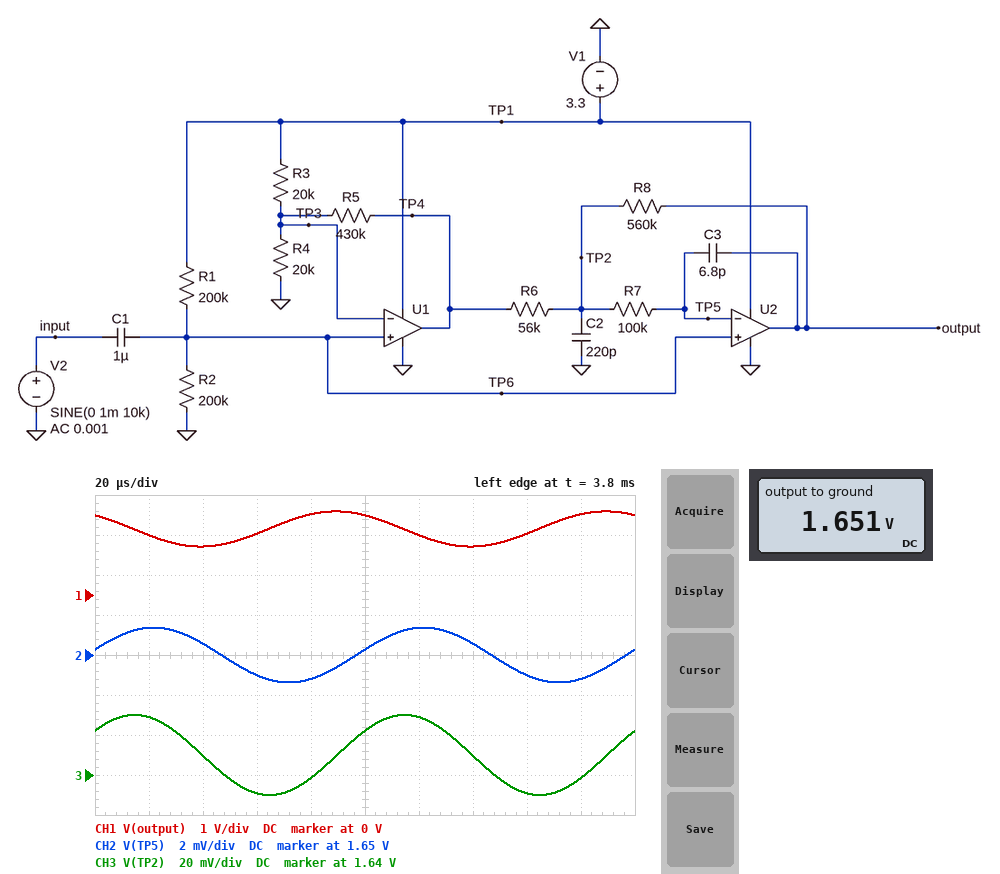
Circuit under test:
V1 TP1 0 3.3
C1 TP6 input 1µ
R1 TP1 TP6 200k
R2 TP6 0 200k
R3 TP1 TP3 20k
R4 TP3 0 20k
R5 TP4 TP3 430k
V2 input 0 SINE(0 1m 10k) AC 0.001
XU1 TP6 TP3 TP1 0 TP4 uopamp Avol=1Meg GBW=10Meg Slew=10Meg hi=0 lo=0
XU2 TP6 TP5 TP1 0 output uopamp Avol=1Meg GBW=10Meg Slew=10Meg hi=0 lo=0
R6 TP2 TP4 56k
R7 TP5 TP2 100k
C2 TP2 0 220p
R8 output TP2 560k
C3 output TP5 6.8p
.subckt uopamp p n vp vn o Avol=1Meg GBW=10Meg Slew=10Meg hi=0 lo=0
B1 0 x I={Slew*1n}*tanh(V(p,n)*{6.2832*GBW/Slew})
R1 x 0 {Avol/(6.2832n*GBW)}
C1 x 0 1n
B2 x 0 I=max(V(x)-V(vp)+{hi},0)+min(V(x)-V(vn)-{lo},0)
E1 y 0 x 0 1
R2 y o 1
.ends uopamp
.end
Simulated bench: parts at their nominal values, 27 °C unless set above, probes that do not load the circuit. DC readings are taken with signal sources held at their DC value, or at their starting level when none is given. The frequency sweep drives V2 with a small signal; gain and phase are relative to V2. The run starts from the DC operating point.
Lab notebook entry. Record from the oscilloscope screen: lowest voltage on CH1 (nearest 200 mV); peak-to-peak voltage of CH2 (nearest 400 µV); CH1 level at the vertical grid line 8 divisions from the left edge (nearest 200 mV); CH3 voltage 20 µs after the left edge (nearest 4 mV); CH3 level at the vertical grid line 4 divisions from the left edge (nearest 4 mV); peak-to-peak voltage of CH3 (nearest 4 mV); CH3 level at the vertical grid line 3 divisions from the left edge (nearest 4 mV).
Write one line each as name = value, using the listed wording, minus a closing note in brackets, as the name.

lowest voltage on CH1 = 1.2 V
peak-to-peak voltage of CH2 = 2.8 mV
CH1 level at the vertical grid line 8 divisions from the left edge = 1.6 V
CH3 voltage 20 µs after the left edge = 1.668 V
CH3 level at the vertical grid line 4 divisions from the left edge = 1.640 V
peak-to-peak voltage of CH3 = 40 mV
CH3 level at the vertical grid line 3 divisions from the left edge = 1.632 V
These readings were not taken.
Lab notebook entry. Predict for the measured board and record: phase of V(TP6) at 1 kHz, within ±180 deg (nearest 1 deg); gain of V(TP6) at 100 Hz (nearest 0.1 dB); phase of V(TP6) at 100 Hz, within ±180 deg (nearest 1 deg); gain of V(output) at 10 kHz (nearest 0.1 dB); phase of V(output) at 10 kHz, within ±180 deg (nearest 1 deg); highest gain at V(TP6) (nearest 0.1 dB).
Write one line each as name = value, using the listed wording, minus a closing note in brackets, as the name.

phase of V(TP6) at 1 kHz, within ±180 deg = 0 deg
gain of V(TP6) at 100 Hz = 0 dB
phase of V(TP6) at 100 Hz, within ±180 deg = 1 deg
gain of V(output) at 10 kHz = 52.9 dB
phase of V(output) at 10 kHz, within ±180 deg = 129 deg
highest gain at V(TP6) = 0 dB
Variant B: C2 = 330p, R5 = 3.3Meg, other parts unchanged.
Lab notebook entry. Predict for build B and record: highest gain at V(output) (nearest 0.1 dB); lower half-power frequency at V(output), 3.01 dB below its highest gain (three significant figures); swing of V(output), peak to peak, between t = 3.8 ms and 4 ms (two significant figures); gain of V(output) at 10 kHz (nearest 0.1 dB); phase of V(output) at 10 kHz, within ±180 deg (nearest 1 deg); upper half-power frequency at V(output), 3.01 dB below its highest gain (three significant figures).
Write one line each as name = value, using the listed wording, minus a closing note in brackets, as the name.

highest gain at V(output) = 71.2 dB
lower half-power frequency at V(output), 3.01 dB below its highest gain = 1.95 Hz
swing of V(output), peak to peak, between t = 3.8 ms and 4 ms = 3.3 V
gain of V(output) at 10 kHz = 71.1 dB
phase of V(output) at 10 kHz, within ±180 deg = 106 deg
upper half-power frequency at V(output), 3.01 dB below its highest gain = 15.6 kHz
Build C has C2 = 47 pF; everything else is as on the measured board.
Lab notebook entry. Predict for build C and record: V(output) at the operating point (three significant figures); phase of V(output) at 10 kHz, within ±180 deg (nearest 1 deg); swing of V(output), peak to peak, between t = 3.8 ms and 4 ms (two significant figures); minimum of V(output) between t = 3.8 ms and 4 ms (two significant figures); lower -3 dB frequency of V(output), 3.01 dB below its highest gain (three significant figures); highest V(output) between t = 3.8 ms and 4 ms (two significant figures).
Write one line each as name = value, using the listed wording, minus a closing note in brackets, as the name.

V(output) at the operating point = 1.65 V
phase of V(output) at 10 kHz, within ±180 deg = 139 deg
swing of V(output), peak to peak, between t = 3.8 ms and 4 ms = 730 mV
minimum of V(output) between t = 3.8 ms and 4 ms = 1.3 V
lower -3 dB frequency of V(output), 3.01 dB below its highest gain = 1.59 Hz
highest V(output) between t = 3.8 ms and 4 ms = 2.0 V
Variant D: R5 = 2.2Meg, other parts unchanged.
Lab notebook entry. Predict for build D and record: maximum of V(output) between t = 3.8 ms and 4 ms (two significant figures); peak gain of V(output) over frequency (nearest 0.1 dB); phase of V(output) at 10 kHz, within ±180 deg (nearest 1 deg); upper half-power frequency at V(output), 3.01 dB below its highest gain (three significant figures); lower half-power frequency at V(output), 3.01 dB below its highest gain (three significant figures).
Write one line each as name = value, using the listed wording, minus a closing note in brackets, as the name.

maximum of V(output) between t = 3.8 ms and 4 ms = 3.3 V
peak gain of V(output) over frequency = 67.0 dB
phase of V(output) at 10 kHz, within ±180 deg = 120 deg
upper half-power frequency at V(output), 3.01 dB below its highest gain = 18.0 kHz
lower half-power frequency at V(output), 3.01 dB below its highest gain = 1.64 Hz
